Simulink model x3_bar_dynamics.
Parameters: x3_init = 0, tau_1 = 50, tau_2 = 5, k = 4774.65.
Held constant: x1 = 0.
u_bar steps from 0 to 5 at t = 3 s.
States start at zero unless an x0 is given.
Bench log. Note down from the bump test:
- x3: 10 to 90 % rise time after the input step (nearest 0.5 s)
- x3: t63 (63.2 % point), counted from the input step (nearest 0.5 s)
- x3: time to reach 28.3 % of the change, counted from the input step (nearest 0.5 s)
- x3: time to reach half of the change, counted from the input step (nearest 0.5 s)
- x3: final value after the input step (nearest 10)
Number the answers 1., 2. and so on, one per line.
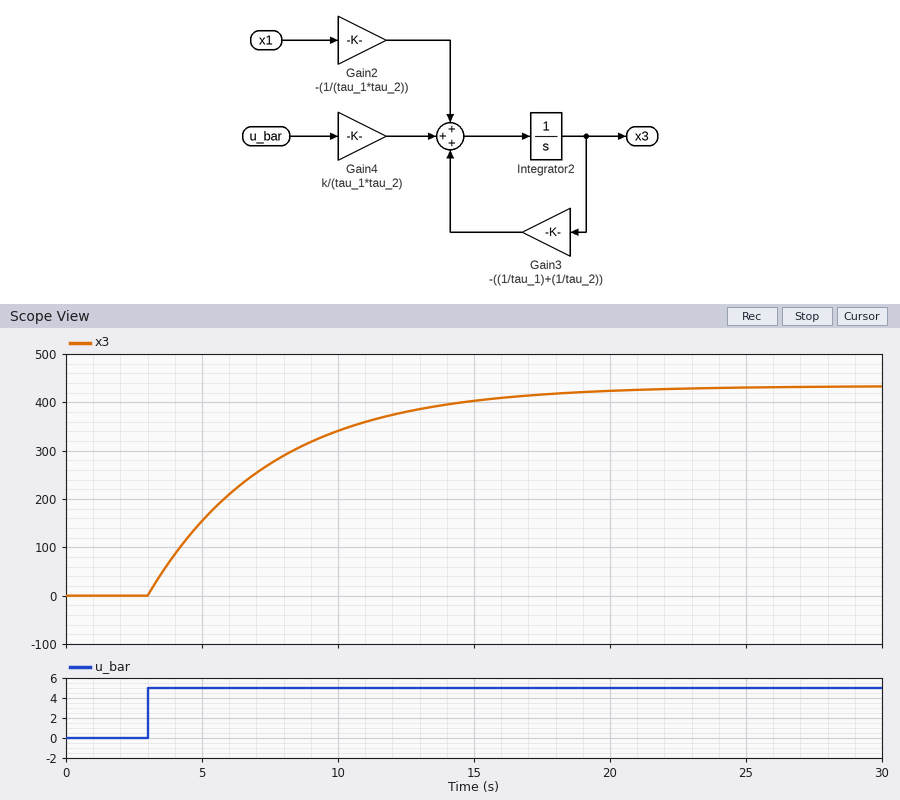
1. 10.0 s
2. 4.5 s
3. 1.5 s
4. 3.0 s
5. 430
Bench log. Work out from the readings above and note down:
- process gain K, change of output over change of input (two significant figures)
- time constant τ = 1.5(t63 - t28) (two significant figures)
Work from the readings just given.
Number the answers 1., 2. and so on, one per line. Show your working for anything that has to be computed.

1. (430 - 0) / 5 = 86
2. 1.5 × (4.5 - 1.5) = 4.5 s
